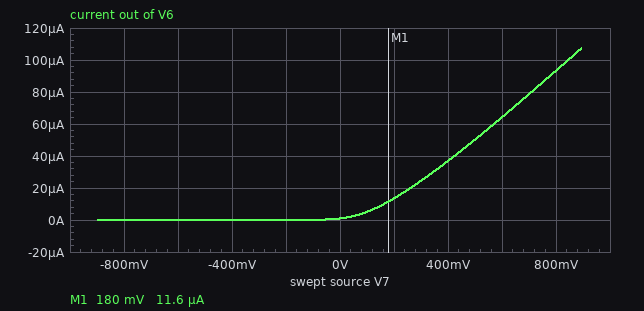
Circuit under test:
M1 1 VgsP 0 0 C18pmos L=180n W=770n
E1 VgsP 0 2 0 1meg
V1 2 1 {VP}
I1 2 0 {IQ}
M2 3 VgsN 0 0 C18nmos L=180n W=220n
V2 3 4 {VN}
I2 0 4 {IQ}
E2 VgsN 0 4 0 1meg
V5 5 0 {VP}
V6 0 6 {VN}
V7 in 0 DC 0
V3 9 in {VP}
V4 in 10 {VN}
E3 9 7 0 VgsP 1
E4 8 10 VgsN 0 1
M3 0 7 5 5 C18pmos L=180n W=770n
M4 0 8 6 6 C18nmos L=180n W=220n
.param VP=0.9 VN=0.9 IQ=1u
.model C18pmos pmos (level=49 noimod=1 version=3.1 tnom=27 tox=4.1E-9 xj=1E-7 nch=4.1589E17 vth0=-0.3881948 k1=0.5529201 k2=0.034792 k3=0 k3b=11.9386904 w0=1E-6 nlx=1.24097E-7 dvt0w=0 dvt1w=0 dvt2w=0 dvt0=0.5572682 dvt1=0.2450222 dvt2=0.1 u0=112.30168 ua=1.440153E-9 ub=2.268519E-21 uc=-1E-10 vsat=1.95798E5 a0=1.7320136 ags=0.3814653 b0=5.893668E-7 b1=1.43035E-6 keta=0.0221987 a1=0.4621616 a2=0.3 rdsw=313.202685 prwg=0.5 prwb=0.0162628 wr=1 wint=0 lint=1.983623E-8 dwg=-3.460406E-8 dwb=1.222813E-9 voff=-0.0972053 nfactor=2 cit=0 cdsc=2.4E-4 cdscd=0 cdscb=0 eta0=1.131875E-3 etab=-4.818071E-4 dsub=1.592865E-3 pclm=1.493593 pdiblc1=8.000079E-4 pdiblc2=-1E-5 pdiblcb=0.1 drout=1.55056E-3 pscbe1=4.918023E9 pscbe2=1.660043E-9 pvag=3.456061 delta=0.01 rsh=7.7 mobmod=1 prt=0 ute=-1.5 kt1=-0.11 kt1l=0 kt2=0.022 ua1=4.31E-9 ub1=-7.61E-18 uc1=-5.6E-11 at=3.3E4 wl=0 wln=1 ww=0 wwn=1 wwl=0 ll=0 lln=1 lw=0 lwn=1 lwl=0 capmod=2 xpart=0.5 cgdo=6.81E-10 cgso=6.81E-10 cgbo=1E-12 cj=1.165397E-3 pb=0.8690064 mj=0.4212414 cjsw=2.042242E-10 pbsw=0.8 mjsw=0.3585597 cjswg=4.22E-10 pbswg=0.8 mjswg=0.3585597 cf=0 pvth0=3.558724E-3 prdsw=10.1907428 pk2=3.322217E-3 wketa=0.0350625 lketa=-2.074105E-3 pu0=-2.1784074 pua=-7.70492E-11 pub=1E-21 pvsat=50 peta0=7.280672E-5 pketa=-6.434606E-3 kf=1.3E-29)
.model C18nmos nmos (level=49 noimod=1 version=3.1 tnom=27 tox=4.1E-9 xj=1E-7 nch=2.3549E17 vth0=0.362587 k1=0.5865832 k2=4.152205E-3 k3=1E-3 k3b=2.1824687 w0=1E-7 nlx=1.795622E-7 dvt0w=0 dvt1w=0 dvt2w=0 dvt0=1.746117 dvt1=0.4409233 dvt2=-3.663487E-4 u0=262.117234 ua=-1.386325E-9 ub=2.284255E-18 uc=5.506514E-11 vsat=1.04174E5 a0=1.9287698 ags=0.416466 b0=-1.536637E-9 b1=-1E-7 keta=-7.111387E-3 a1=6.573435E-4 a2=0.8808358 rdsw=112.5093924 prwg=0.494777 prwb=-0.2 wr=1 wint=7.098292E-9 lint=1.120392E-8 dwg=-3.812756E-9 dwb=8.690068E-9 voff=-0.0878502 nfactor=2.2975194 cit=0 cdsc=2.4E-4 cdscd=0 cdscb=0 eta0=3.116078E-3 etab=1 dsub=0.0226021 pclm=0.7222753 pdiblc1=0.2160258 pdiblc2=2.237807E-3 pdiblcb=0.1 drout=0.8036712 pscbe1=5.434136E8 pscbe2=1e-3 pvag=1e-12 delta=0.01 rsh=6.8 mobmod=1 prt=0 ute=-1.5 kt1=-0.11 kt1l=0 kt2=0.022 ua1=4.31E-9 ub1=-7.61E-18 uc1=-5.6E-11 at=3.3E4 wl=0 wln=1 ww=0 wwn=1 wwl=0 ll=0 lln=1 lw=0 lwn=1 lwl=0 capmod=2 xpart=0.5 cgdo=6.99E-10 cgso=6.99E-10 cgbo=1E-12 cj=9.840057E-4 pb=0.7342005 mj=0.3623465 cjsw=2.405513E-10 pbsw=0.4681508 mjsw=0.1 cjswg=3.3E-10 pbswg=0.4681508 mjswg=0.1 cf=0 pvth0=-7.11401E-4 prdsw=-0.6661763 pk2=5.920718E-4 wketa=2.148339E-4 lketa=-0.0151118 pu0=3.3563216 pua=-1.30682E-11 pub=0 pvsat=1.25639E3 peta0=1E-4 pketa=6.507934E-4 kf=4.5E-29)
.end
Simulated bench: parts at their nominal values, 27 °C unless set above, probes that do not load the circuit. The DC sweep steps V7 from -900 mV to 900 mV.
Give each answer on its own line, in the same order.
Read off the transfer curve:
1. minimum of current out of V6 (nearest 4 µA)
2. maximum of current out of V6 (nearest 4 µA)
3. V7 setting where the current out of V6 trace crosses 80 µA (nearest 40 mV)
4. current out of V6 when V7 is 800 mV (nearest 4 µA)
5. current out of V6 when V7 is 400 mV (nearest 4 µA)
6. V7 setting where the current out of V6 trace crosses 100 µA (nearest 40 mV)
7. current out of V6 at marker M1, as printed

0 A
108 µA
720 mV
92 µA
36 µA
840 mV
11.6 µA
